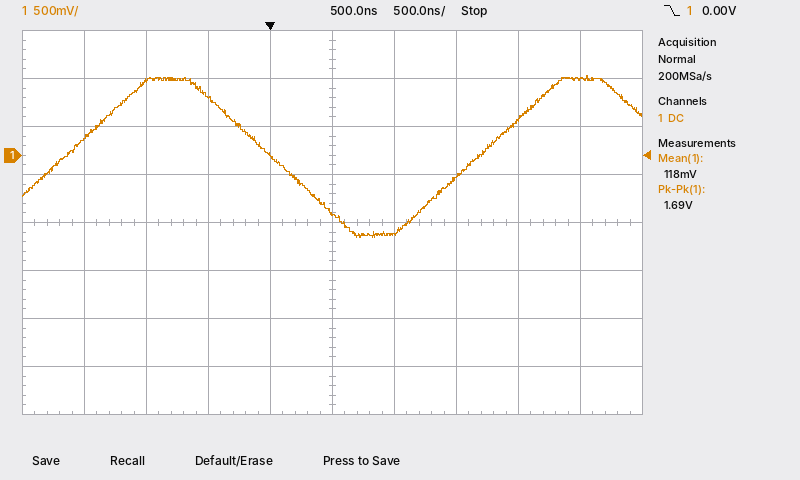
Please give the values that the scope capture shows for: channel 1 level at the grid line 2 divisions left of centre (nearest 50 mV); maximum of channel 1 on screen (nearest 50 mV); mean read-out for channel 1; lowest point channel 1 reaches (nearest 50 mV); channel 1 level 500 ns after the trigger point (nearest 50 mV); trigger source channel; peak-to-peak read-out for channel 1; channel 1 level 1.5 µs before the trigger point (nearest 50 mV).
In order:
600 mV
850 mV
118 mV
-850 mV
-600 mV
channel 1
1.69 V
200 mV
